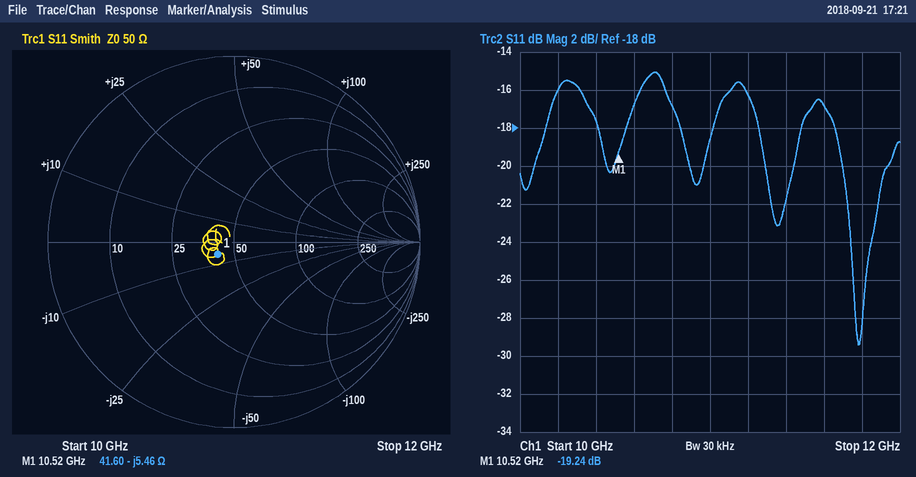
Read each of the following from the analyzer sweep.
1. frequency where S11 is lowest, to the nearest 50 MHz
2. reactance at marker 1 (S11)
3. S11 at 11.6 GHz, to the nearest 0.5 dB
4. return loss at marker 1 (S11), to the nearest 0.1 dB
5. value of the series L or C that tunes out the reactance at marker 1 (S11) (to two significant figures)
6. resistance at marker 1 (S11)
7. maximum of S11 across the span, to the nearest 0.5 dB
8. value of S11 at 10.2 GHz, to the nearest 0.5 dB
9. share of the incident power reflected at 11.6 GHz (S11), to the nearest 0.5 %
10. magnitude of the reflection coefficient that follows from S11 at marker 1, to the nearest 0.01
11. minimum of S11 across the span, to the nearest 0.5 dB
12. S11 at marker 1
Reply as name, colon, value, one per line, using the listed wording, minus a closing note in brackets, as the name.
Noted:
frequency where S11 is lowest, to the nearest 50 MHz: 11.80 GHz
reactance at marker 1: -5.46 Ω
S11 at 11.6 GHz, to the nearest 0.5 dB: -17.0 dB
return loss at marker 1 (S11), to the nearest 0.1 dB: 19.2 dB
value of the series L or C that tunes out the reactance at marker 1 (S11): 83 pH
resistance at marker 1: 41.60 Ω
maximum of S11 across the span, to the nearest 0.5 dB: -15.0 dB
value of S11 at 10.2 GHz, to the nearest 0.5 dB: -16.0 dB
share of the incident power reflected at 11.6 GHz (S11), to the nearest 0.5 %: 2.0 %
magnitude of the reflection coefficient that follows from S11 at marker 1, to the nearest 0.01: 0.11
minimum of S11 across the span, to the nearest 0.5 dB: -29.5 dB
S11 at marker 1: -19.24 dB
